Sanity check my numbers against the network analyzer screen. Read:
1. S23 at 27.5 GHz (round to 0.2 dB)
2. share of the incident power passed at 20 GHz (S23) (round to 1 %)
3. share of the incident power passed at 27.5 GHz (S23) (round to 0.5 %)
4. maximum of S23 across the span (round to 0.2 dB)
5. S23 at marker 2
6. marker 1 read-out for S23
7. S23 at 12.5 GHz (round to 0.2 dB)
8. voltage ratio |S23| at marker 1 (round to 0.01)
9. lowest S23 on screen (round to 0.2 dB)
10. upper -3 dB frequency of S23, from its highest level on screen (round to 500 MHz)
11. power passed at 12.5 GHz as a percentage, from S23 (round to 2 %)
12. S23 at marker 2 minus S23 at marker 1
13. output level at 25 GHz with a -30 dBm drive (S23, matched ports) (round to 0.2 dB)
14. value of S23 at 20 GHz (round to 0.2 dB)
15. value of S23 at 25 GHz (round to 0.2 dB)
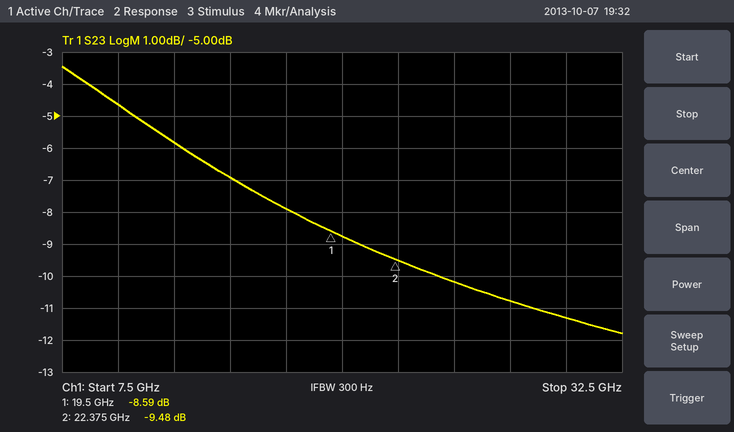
-10.8 dB
13 %
8.5 %
-3.4 dB
-9.48 dB
-8.59 dB
-5.8 dB
0.37
-11.8 dB
14.0 GHz
26 %
-0.89 dB
-40.2 dBm
-8.8 dB
-10.2 dB
